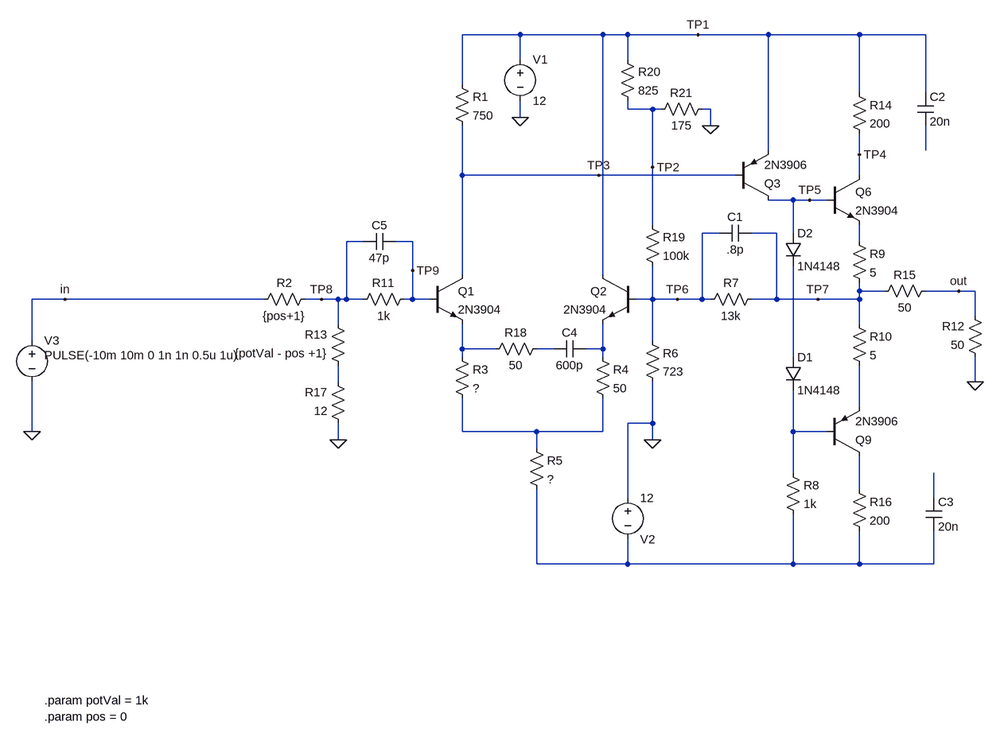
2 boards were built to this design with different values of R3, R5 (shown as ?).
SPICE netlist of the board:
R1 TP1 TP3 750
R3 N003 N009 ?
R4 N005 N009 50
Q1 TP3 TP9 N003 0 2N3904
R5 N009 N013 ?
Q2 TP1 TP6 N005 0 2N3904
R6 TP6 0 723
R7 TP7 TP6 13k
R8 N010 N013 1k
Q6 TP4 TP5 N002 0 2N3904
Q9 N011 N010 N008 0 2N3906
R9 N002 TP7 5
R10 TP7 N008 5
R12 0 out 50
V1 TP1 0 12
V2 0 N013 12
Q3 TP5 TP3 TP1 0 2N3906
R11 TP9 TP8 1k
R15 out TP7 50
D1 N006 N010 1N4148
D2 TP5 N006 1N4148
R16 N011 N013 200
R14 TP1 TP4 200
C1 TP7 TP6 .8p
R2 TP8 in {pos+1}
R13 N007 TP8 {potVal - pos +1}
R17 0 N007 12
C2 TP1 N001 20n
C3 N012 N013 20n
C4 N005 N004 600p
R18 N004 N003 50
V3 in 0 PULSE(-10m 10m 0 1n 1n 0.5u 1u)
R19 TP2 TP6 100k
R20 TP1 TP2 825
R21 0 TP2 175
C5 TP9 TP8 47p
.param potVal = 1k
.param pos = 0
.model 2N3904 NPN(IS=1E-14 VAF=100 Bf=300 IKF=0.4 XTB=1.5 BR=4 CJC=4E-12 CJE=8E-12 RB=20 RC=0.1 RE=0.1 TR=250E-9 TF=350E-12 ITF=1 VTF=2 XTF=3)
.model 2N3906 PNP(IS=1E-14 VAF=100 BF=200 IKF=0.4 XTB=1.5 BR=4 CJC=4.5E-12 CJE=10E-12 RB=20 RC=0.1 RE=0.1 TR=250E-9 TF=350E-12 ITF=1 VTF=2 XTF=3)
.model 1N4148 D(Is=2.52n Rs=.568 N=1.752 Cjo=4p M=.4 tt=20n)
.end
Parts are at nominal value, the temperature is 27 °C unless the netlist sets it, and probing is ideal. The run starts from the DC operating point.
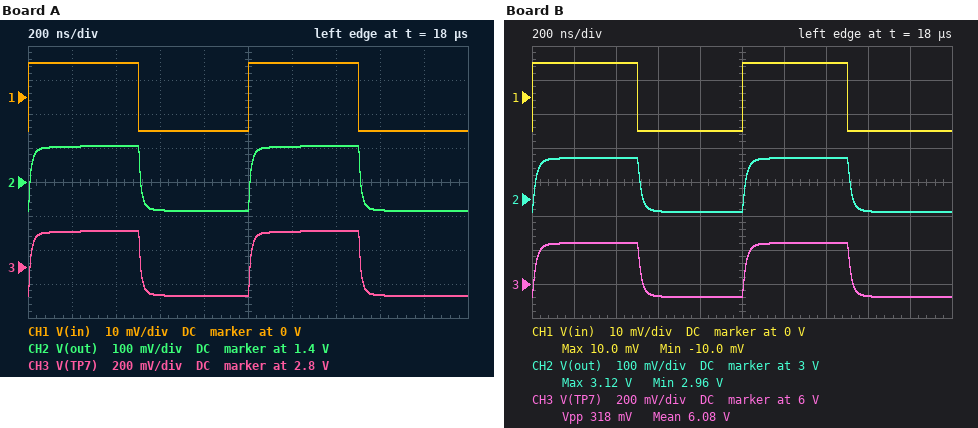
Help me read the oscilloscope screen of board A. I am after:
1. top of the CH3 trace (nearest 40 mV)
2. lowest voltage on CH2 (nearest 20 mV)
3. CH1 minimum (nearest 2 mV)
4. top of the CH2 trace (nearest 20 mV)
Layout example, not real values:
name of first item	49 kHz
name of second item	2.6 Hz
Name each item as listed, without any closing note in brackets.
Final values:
top of the CH3 trace	3.00 V
lowest voltage on CH2	1.32 V
CH1 minimum	-10 mV
top of the CH2 trace	1.50 V
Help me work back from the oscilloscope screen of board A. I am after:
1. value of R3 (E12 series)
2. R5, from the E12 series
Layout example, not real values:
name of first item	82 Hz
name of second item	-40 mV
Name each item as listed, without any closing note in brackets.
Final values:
value of R3	27 Ω
R5, from the E12 series	2.7 kΩ
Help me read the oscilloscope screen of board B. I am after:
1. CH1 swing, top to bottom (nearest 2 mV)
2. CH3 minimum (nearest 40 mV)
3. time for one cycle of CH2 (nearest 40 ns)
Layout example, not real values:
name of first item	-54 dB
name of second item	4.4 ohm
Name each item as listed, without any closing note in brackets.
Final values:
CH1 swing, top to bottom	20 mV
CH3 minimum	5.92 V
time for one cycle of CH2	1.00 µs
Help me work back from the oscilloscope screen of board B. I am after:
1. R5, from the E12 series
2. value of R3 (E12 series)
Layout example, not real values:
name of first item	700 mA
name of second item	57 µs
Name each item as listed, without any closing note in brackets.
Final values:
R5, from the E12 series	1.5 kΩ
value of R3	22 Ω
